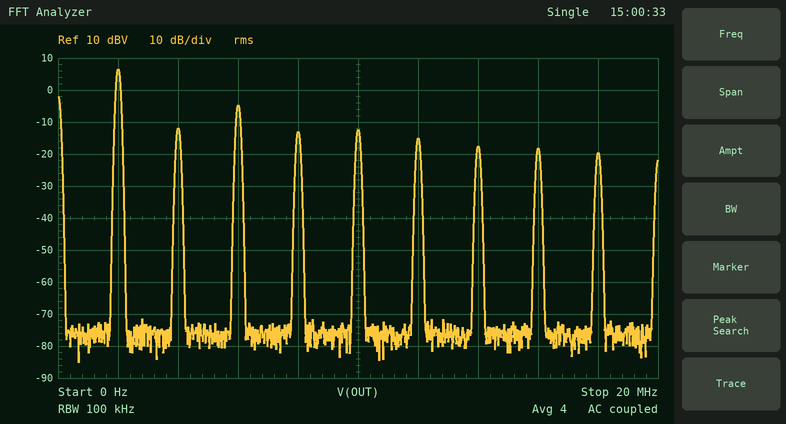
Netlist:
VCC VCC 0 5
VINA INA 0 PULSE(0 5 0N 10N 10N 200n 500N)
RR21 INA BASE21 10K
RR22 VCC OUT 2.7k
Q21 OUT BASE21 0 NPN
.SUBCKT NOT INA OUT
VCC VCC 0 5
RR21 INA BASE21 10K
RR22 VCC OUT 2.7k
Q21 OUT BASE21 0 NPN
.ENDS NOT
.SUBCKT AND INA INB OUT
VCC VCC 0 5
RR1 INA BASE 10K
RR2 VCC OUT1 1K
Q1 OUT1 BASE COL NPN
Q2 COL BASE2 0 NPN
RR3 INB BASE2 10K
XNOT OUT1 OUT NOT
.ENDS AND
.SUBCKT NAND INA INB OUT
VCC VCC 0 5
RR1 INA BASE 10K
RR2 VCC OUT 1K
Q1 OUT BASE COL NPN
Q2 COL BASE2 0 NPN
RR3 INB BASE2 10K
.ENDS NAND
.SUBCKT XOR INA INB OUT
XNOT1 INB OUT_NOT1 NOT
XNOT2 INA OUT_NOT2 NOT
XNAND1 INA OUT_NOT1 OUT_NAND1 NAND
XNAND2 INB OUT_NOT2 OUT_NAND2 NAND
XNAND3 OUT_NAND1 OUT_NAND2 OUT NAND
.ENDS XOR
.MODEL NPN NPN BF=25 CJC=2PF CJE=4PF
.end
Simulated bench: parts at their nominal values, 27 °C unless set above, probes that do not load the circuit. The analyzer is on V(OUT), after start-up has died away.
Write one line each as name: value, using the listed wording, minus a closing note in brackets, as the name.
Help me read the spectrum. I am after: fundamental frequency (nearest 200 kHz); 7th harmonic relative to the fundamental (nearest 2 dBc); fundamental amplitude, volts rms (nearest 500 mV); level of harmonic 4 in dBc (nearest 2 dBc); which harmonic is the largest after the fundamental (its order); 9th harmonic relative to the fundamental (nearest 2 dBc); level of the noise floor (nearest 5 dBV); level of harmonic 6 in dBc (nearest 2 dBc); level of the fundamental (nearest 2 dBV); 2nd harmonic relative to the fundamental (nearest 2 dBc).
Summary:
fundamental frequency: 2.0 MHz
7th harmonic relative to the fundamental: -24 dBc
fundamental amplitude, volts rms: 2.0 V
level of harmonic 4 in dBc: -20 dBc
which harmonic is the largest after the fundamental: 3
9th harmonic relative to the fundamental: -26 dBc
level of the noise floor: -75 dBV
level of harmonic 6 in dBc: -22 dBc
level of the fundamental: 6 dBV
2nd harmonic relative to the fundamental: -18 dBc
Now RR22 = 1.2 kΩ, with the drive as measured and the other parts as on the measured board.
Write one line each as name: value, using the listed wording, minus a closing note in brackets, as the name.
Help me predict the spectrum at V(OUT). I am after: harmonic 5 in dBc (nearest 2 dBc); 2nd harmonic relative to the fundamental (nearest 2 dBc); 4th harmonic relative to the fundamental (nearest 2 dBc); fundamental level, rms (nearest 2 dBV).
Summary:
harmonic 5 in dBc: -22 dBc
2nd harmonic relative to the fundamental: -14 dBc
4th harmonic relative to the fundamental: -16 dBc
fundamental level, rms: 6 dBV
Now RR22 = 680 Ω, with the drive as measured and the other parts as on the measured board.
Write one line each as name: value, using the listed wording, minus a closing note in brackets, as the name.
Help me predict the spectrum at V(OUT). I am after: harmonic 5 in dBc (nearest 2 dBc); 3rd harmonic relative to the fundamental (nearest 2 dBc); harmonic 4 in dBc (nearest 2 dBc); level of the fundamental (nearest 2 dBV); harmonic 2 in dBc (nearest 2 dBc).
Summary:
harmonic 5 in dBc: -30 dBc
3rd harmonic relative to the fundamental: -14 dBc
harmonic 4 in dBc: -14 dBc
level of the fundamental: 6 dBV
harmonic 2 in dBc: -12 dBc
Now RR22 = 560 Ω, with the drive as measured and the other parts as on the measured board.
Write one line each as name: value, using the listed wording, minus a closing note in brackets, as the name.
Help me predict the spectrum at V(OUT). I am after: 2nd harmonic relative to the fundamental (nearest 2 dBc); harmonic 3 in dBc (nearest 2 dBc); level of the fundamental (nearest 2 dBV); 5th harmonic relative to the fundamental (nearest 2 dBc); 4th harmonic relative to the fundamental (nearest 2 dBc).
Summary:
2nd harmonic relative to the fundamental: -10 dBc
harmonic 3 in dBc: -14 dBc
level of the fundamental: 6 dBV
5th harmonic relative to the fundamental: -38 dBc
4th harmonic relative to the fundamental: -14 dBc
